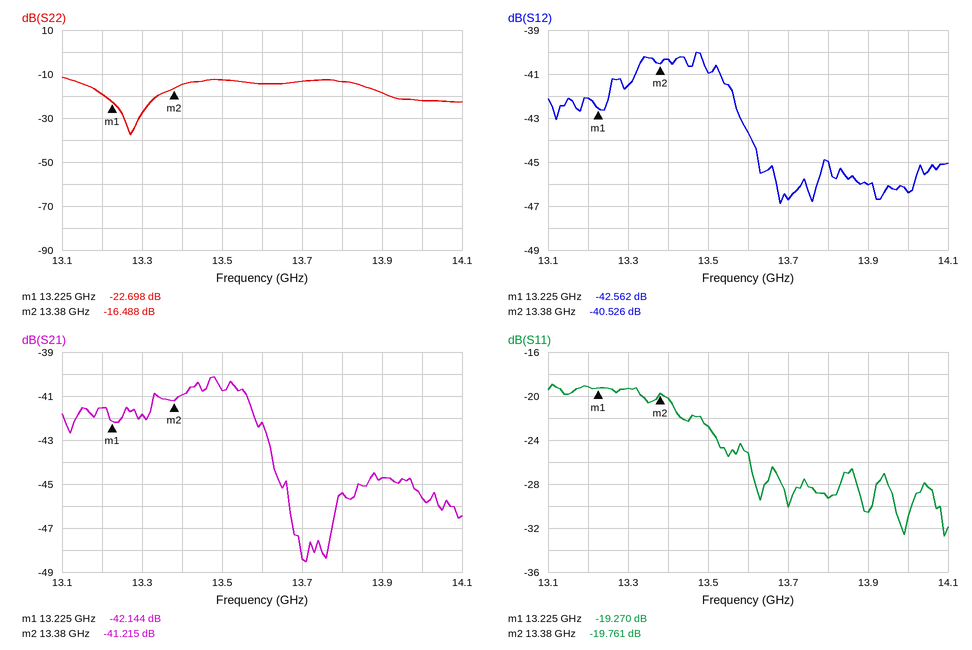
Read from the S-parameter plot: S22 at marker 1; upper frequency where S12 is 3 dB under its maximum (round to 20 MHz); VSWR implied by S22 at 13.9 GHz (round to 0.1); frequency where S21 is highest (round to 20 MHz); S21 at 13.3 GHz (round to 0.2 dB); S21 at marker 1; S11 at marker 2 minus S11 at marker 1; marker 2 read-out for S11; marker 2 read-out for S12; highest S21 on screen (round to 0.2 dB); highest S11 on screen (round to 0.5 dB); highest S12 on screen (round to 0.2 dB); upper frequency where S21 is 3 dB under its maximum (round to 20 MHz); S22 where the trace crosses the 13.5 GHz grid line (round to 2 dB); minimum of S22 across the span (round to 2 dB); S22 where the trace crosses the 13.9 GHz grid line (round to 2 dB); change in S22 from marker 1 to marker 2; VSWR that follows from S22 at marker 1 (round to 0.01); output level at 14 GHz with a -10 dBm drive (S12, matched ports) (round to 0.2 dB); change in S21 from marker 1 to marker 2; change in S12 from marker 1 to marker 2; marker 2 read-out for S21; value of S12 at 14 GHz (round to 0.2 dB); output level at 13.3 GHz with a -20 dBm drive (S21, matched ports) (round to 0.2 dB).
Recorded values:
-22.698 dB
13.58 GHz
1.3
13.48 GHz
-41.8 dB
-42.144 dB
-0.491 dB
-19.761 dB
-40.526 dB
-40.2 dB
-19.0 dB
-40.0 dB
13.62 GHz
-12 dB
-38 dB
-18 dB
6.210 dB
1.16
-56.4 dBm
0.929 dB
2.036 dB
-41.215 dB
-46.4 dB
-61.8 dBm
